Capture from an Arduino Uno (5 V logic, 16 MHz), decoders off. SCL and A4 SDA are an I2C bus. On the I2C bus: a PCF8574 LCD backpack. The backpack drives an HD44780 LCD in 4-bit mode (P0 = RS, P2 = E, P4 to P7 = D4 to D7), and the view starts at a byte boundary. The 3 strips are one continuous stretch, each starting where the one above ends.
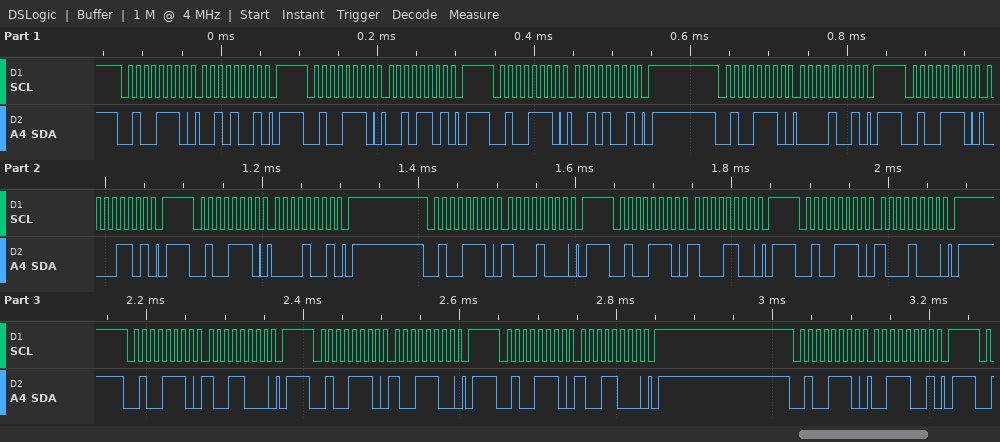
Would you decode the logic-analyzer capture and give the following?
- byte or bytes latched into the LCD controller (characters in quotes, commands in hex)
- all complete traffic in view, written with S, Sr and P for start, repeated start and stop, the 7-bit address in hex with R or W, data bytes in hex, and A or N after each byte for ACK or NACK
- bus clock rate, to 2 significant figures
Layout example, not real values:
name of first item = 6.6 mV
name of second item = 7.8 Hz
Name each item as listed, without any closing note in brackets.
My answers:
byte or bytes latched into the LCD controller = ' ' 0x89
all complete traffic in view, written with S, Sr and P for start, repeated start and stop, the 7-bit address in hex with R or W, data bytes in hex, and A or N after each byte for ACK or NACK = S 27W A 29 A P S 27W A 2D A P S 27W A 29 A P S 27W A 09 A P S 27W A 0D A P S 27W A 09 A P S 27W A 88 A P S 27W A 8C A P S 27W A 88 A P S 27W A 98 A P S 27W A 9C A P S 27W A 98 A P S 27W A 39 A P
bus clock rate, to 2 significant figures = 100 kHz
